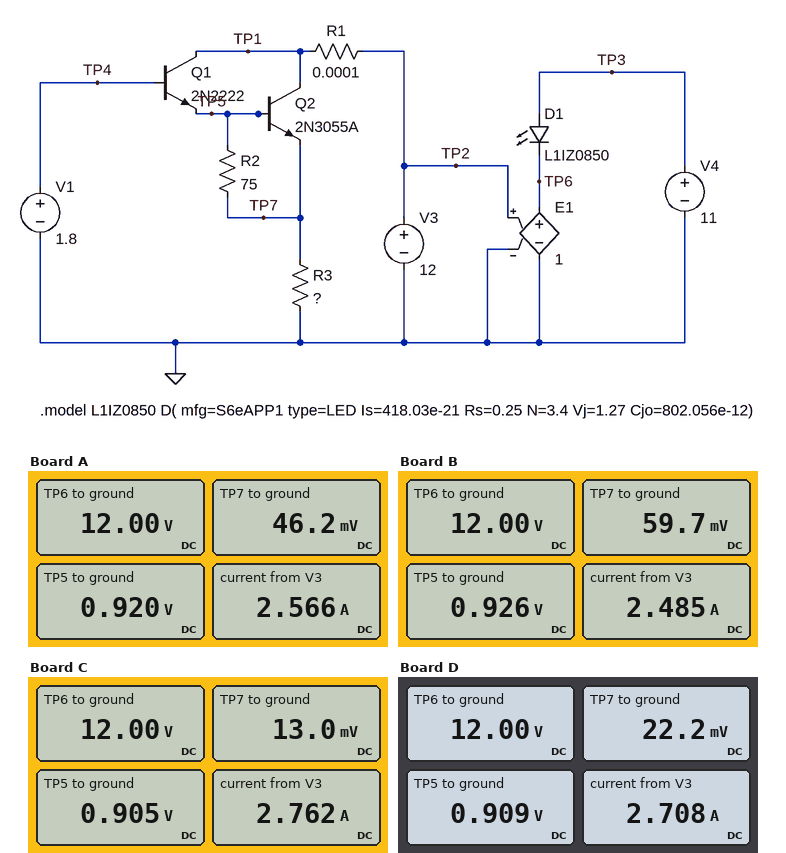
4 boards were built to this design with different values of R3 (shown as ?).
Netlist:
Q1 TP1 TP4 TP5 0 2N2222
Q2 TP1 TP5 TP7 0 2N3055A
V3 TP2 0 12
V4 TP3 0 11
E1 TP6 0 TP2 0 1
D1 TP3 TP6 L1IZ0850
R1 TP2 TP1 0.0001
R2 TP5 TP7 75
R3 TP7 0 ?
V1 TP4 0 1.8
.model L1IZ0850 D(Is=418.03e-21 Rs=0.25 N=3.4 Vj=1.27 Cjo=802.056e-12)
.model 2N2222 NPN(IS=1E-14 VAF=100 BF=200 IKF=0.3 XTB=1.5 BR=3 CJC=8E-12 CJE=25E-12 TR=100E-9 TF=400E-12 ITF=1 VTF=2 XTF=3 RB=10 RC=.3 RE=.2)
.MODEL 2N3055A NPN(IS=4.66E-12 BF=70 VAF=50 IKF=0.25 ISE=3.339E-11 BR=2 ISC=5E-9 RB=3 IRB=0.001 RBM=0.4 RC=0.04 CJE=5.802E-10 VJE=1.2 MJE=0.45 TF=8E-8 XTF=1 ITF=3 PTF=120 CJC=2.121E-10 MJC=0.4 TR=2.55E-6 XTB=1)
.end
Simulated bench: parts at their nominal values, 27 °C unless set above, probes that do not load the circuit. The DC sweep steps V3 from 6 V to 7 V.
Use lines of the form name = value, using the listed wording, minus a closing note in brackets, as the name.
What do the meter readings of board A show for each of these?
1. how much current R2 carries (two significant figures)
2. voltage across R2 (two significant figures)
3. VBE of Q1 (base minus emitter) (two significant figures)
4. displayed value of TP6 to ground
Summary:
how much current R2 carries = 12 mA
voltage across R2 = 870 mV
VBE of Q1 (base minus emitter) = 880 mV
displayed value of TP6 to ground = 12.00 V
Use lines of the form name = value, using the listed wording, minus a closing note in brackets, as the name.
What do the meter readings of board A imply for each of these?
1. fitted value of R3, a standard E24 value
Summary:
fitted value of R3, a standard E24 value = 0.018 Ω
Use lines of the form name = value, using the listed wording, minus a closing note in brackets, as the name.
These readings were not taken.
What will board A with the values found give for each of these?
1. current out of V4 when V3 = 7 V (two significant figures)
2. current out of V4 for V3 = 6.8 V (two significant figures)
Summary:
current out of V4 when V3 = 7 V = 1.1 A
current out of V4 for V3 = 6.8 V = 1.7 A
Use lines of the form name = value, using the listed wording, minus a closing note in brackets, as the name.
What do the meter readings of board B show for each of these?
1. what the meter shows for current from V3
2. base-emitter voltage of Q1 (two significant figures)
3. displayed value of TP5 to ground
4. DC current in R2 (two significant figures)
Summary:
what the meter shows for current from V3 = 2.485 A
base-emitter voltage of Q1 = 870 mV
displayed value of TP5 to ground = 0.926 V
DC current in R2 = 12 mA
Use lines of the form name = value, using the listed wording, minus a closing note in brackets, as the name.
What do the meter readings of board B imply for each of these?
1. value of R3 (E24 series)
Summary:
value of R3 = 0.024 Ω
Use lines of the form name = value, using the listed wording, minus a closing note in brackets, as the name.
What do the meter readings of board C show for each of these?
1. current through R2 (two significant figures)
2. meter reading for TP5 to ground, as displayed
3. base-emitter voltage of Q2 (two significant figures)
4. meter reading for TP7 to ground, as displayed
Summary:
current through R2 = 12 mA
meter reading for TP5 to ground, as displayed = 0.905 V
base-emitter voltage of Q2 = 890 mV
meter reading for TP7 to ground, as displayed = 13.0 mV
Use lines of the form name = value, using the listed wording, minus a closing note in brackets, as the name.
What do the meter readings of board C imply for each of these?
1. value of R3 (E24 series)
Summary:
value of R3 = 4.7 mΩ
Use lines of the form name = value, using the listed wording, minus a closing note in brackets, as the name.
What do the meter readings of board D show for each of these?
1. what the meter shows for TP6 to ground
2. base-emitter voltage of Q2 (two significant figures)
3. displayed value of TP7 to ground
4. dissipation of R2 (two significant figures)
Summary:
what the meter shows for TP6 to ground = 12.00 V
base-emitter voltage of Q2 = 890 mV
displayed value of TP7 to ground = 22.2 mV
dissipation of R2 = 10 mW
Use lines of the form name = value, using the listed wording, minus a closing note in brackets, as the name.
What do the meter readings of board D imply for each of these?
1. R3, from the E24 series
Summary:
R3, from the E24 series = 8.2 mΩ
